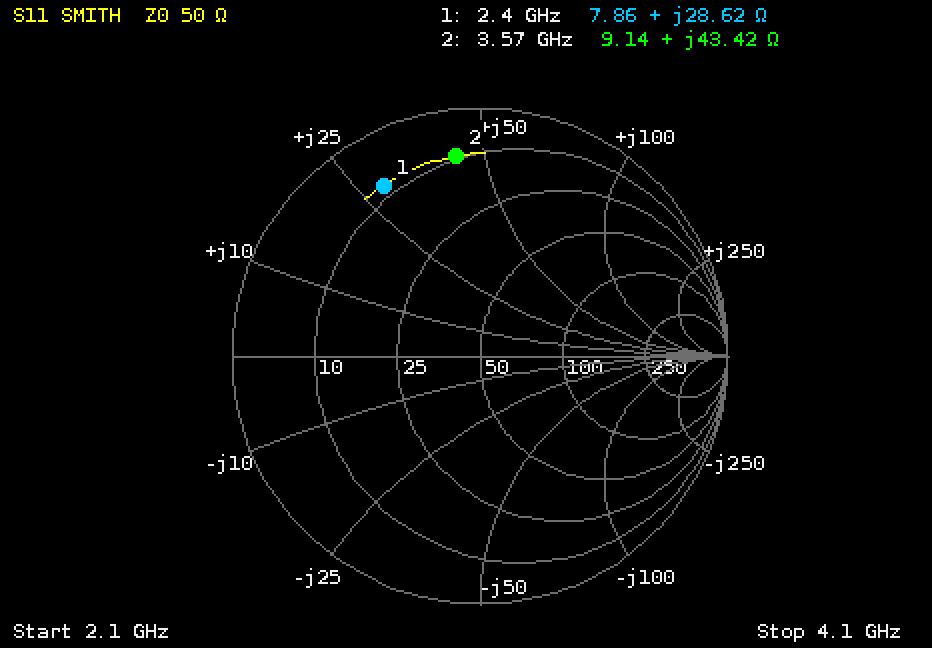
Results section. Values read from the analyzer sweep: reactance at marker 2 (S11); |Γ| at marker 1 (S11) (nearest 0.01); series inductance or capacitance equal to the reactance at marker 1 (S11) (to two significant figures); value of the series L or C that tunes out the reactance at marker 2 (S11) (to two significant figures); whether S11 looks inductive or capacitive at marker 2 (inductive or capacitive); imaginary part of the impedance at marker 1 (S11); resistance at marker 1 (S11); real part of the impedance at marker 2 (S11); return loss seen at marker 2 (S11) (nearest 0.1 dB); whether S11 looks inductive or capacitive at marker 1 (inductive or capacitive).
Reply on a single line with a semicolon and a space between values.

+43.42 Ω; 0.79; 1.9 nH; 1.0 pF; inductive; +28.62 Ω; 7.86 Ω; 9.14 Ω; 1.8 dB; inductive
